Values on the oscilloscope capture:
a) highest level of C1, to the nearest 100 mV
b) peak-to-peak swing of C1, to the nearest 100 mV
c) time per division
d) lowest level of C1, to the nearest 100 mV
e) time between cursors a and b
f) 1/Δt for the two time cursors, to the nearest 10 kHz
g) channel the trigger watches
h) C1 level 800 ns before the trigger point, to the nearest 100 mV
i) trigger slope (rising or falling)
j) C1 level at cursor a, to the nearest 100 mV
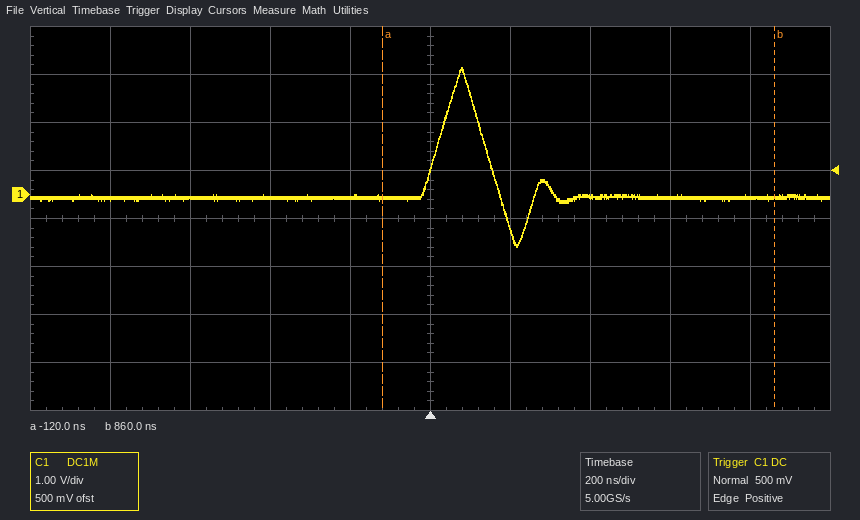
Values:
2.6 V
3.7 V
200 ns
-1.1 V
980 ns
1.02 MHz
C1
-100 mV
rising
-100 mV
